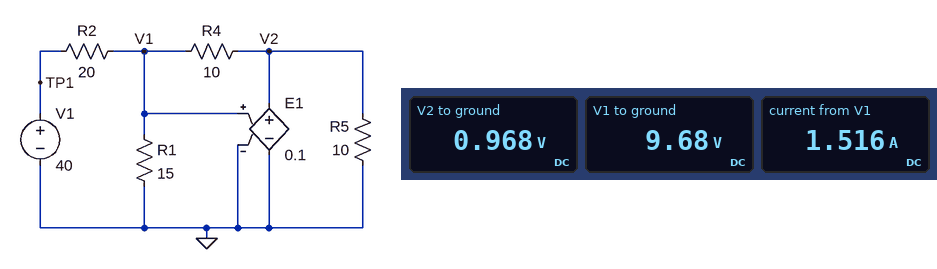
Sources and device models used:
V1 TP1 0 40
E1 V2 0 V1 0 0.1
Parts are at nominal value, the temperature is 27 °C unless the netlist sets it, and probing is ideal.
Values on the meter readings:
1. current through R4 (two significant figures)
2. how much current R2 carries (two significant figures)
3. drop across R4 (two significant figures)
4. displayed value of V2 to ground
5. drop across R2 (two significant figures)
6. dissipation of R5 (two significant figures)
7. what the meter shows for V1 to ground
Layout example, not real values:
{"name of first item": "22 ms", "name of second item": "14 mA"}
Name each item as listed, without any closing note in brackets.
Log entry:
{"current through R4": "870 mA", "how much current R2 carries": "1.5 A", "drop across R4": "8.7 V", "displayed value of V2 to ground": "0.968 V", "drop across R2": "30 V", "dissipation of R5": "94 mW", "what the meter shows for V1 to ground": "9.68 V"}
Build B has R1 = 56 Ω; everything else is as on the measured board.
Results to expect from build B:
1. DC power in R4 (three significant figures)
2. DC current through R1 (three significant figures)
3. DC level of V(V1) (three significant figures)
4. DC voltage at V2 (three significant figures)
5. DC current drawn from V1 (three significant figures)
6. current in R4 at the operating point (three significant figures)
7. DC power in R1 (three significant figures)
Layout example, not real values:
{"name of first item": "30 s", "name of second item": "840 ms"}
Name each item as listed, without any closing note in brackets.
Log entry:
{"DC power in R4": "13.0 W", "DC current through R1": "226 mA", "DC level of V(V1)": "12.7 V", "DC voltage at V2": "1.27 V", "DC current drawn from V1": "1.37 A", "current in R4 at the operating point": "1.14 A", "DC power in R1": "2.87 W"}
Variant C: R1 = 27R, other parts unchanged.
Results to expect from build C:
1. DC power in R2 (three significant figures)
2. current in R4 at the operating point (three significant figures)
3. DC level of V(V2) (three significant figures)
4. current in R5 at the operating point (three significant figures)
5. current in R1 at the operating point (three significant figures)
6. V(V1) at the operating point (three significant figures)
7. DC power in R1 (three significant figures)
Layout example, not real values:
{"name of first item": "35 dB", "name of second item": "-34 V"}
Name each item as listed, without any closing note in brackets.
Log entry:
{"DC power in R2": "41.2 W", "current in R4 at the operating point": "1.02 A", "DC level of V(V2)": "1.13 V", "current in R5 at the operating point": "113 mA", "current in R1 at the operating point": "418 mA", "V(V1) at the operating point": "11.3 V", "DC power in R1": "4.73 W"}
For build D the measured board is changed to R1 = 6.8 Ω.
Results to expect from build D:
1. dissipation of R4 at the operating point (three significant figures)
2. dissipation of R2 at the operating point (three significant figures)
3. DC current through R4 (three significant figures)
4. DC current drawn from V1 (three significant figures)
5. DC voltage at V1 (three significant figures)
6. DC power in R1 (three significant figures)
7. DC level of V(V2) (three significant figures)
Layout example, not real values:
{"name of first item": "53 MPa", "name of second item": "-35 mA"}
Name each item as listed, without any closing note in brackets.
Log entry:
{"dissipation of R4 at the operating point": "3.93 W", "dissipation of R2 at the operating point": "54.6 W", "DC current through R4": "627 mA", "DC current drawn from V1": "1.65 A", "DC voltage at V1": "6.97 V", "DC power in R1": "7.14 W", "DC level of V(V2)": "697 mV"}
